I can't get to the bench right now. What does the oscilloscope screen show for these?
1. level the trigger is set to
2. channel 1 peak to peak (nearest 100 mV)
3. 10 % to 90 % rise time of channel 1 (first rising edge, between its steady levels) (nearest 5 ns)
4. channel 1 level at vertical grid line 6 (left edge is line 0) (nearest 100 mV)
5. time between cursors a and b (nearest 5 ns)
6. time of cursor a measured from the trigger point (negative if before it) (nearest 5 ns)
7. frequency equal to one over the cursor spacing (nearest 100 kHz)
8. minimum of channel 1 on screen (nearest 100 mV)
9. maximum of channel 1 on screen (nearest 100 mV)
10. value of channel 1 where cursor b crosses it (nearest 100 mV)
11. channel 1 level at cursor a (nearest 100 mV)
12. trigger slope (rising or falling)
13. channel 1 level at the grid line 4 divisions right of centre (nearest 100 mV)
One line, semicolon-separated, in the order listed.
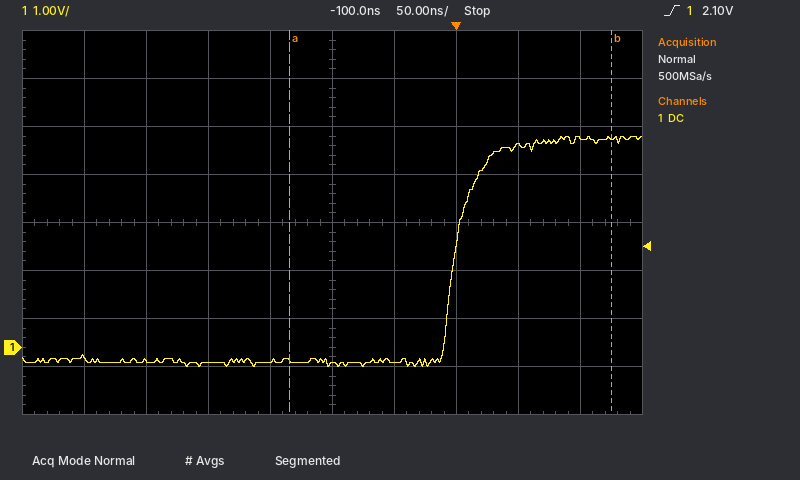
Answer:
2.10 V; 4.8 V; 35 ns; -300 mV; 260 ns; -135 ns; 3.8 MHz; -400 mV; 4.4 V; 4.4 V; -300 mV; rising; 4.4 V
